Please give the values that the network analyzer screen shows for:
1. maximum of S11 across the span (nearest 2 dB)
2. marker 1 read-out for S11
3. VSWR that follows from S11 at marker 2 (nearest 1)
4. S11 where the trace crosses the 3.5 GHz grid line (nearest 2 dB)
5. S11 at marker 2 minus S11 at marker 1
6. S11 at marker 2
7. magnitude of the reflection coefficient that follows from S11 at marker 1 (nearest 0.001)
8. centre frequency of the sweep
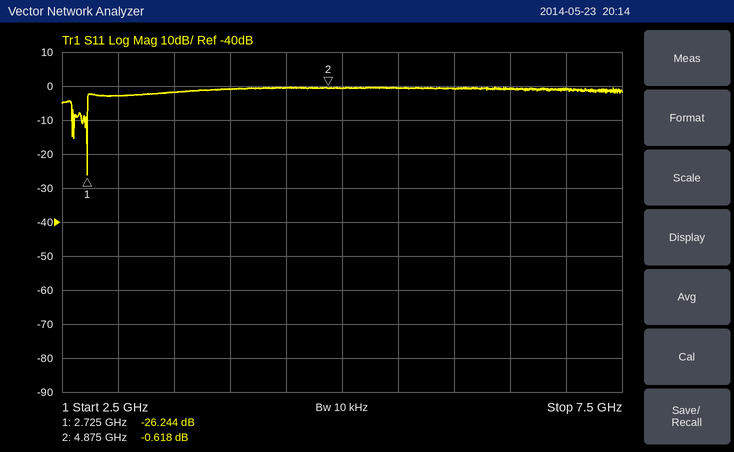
0 dB
-26.244 dB
28
-2 dB
25.626 dB
-0.618 dB
0.049
5 GHz
